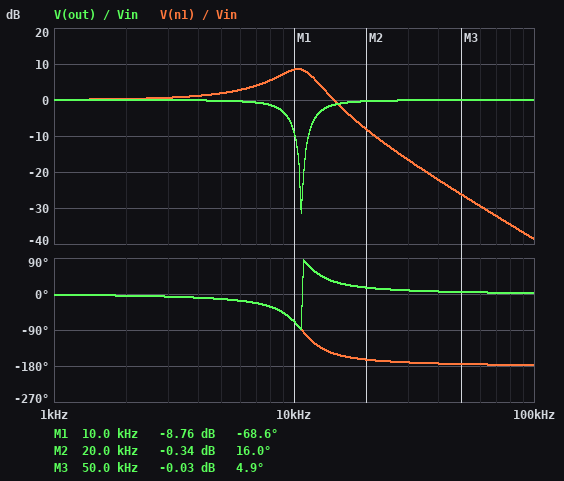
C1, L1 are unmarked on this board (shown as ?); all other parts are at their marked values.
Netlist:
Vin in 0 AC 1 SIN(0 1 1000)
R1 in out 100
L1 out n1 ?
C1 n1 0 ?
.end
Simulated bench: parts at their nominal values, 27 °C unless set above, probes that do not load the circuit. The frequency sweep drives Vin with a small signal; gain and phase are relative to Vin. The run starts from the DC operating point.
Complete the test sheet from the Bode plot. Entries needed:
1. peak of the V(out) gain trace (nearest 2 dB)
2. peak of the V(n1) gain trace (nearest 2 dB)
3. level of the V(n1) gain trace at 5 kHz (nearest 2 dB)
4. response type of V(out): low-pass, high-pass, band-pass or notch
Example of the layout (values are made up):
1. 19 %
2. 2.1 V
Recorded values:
1. 0 dB
2. 8 dB
3. 2 dB
4. notch
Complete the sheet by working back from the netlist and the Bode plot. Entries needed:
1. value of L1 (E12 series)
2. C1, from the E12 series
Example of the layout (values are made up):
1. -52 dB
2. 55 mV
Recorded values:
1. 3.9 mH
2. 56 nF
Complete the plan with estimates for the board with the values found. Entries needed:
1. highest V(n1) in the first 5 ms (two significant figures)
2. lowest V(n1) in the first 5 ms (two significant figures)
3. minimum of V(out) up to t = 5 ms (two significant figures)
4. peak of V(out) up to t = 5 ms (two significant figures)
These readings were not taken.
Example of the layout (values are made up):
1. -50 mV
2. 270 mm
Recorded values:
1. 1.0 V
2. -1.0 V
3. -1.0 V
4. 1.0 V
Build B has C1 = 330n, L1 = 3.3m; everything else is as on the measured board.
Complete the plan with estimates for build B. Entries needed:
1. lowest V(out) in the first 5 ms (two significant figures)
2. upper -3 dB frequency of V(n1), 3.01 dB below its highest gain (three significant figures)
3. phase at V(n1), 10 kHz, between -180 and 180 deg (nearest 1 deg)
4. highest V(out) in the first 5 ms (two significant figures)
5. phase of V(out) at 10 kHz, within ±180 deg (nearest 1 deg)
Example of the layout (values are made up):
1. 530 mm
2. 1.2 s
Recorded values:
1. -980 mV
2. 5.64 kHz
3. -148 deg
4. 980 mV
5. 32 deg
